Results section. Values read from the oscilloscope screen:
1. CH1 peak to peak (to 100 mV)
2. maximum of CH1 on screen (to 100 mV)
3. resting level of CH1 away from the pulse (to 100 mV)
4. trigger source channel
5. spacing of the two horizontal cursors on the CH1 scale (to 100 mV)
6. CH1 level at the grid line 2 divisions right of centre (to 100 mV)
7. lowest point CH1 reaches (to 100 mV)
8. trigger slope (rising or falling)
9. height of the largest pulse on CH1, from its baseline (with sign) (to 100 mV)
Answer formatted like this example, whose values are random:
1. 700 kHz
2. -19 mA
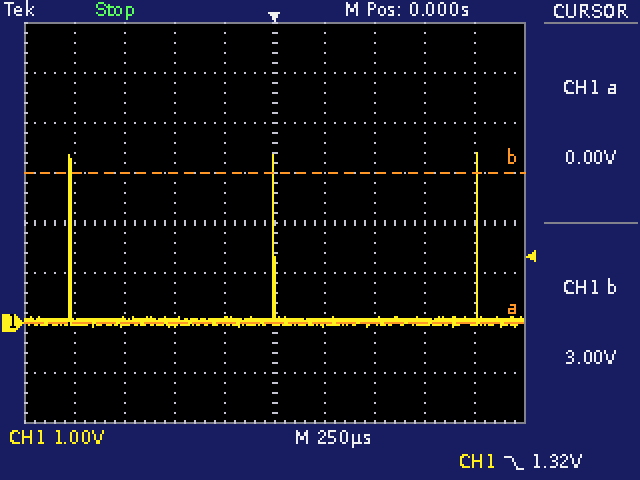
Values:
1. 3.5 V
2. 3.4 V
3. 0.0 V
4. CH1
5. 3.0 V
6. 0.0 V
7. -100 mV
8. falling
9. +3.4 V
